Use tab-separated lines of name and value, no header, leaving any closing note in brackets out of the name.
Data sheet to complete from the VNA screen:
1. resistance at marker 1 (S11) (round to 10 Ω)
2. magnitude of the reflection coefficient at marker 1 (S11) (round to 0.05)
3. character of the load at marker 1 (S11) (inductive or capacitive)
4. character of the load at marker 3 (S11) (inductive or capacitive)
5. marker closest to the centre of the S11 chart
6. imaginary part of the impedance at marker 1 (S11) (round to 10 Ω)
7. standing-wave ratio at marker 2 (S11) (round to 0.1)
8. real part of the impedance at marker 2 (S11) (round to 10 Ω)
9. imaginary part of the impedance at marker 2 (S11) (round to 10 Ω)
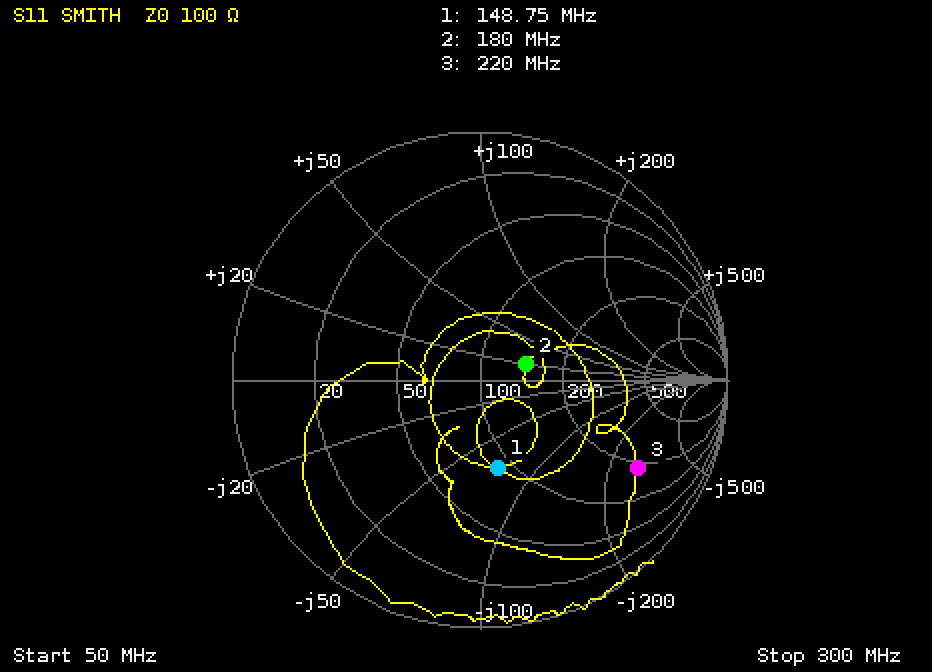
resistance at marker 1 (S11)	90 Ω
magnitude of the reflection coefficient at marker 1 (S11)	0.35
character of the load at marker 1 (S11)	capacitive
character of the load at marker 3 (S11)	capacitive
marker closest to the centre of the S11 chart	marker 2
imaginary part of the impedance at marker 1 (S11)	-70 Ω
standing-wave ratio at marker 2 (S11)	1.5
real part of the impedance at marker 2 (S11)	140 Ω
imaginary part of the impedance at marker 2 (S11)	+20 Ω
